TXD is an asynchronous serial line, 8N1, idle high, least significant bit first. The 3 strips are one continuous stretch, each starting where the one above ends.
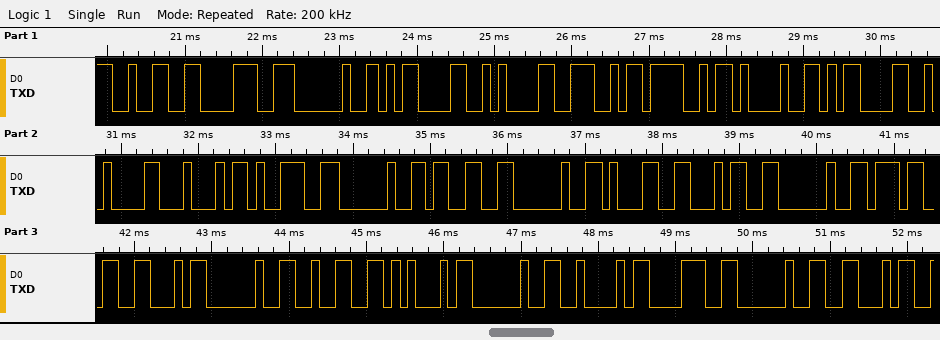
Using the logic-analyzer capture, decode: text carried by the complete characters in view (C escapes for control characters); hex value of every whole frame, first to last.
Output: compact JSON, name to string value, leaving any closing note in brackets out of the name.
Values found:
{"text carried by the complete characters in view": "\"28 \\r\\nNO!\\r\\nD9 3 14 7F 2E B8 F\"", "hex value of every whole frame, first to last": "32 38 20 0D 0A 4E 4F 21 0D 0A 44 39 20 33 20 31 34 20 37 46 20 32 45 20 42 38 20 46"}
